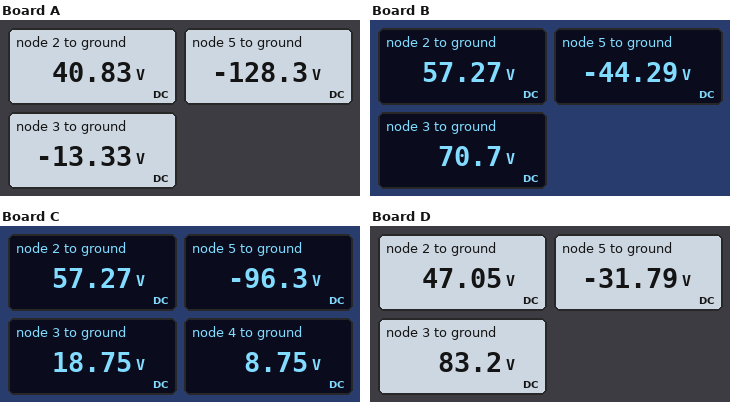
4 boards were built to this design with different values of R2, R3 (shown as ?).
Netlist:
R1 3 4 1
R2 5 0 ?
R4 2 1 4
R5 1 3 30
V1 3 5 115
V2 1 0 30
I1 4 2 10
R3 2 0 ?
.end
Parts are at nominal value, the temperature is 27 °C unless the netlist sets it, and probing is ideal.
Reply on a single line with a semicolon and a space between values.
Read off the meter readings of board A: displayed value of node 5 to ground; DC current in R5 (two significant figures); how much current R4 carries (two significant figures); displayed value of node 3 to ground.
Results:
-128.3 V; 1.4 A; 2.7 A; -13.33 V
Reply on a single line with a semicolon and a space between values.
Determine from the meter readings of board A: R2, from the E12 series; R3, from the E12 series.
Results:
15 Ω; 5.6 Ω
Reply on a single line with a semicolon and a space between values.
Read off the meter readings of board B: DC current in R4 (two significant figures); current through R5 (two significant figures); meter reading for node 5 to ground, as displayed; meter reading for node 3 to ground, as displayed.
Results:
6.8 A; 1.4 A; -44.29 V; 70.7 V
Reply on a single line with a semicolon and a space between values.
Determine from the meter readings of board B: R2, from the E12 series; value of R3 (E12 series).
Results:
3.9 Ω; 18 Ω
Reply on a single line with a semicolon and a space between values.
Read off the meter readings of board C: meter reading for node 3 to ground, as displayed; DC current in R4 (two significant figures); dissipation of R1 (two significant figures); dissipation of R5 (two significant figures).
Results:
18.75 V; 6.8 A; 100 W; 4.2 W
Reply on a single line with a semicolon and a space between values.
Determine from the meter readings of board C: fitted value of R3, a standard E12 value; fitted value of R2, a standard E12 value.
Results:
18 Ω; 10 Ω
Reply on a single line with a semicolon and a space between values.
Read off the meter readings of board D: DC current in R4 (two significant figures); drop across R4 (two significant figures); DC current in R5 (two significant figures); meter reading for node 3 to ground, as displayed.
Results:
4.3 A; 17 V; 1.8 A; 83.2 V
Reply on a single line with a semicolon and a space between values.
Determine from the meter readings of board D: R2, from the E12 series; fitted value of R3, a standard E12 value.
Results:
2.7 Ω; 8.2 Ω
